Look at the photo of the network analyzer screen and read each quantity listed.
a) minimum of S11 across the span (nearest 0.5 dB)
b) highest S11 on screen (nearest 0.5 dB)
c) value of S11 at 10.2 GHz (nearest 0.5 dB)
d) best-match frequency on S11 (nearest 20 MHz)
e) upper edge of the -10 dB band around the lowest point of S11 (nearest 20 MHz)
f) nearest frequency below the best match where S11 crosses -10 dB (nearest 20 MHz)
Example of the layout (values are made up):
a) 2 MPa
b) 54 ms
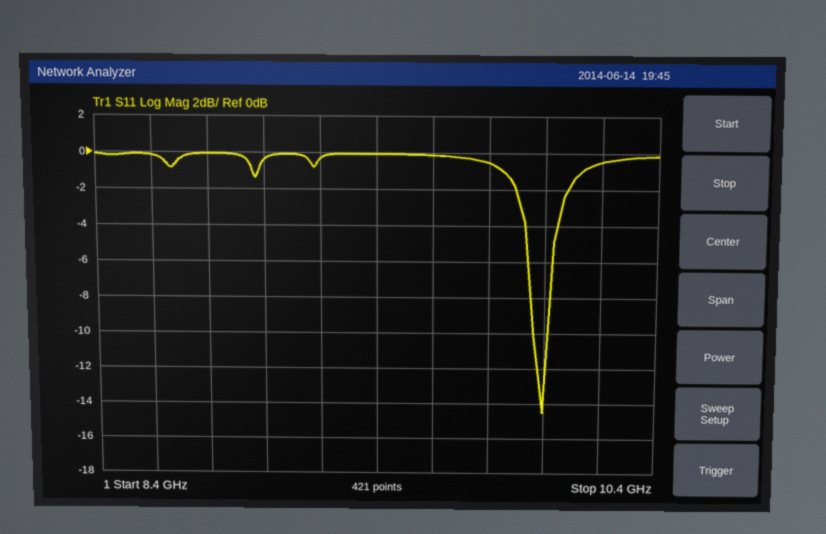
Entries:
a) -14.5 dB
b) 0.0 dB
c) -0.5 dB
d) 10.00 GHz
e) 10.02 GHz
f) 9.96 GHz
